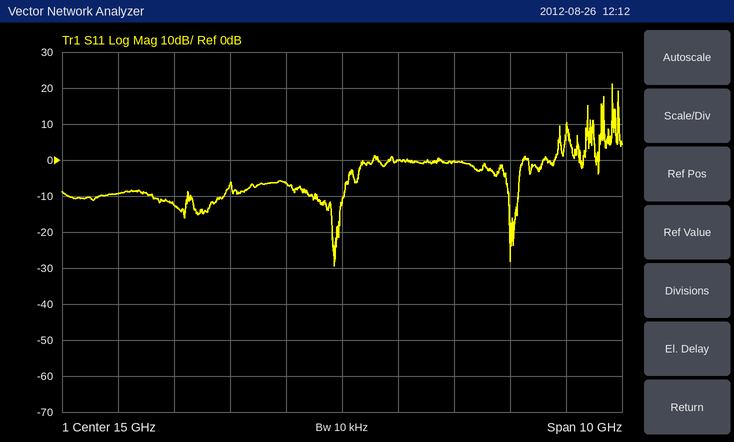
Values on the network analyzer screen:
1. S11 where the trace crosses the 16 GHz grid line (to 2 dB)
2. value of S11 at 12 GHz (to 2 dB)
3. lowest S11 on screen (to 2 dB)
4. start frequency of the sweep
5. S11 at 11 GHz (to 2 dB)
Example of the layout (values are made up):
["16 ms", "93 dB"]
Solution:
["0 dB", "-12 dB", "-30 dB", "10 GHz", "-10 dB"]
